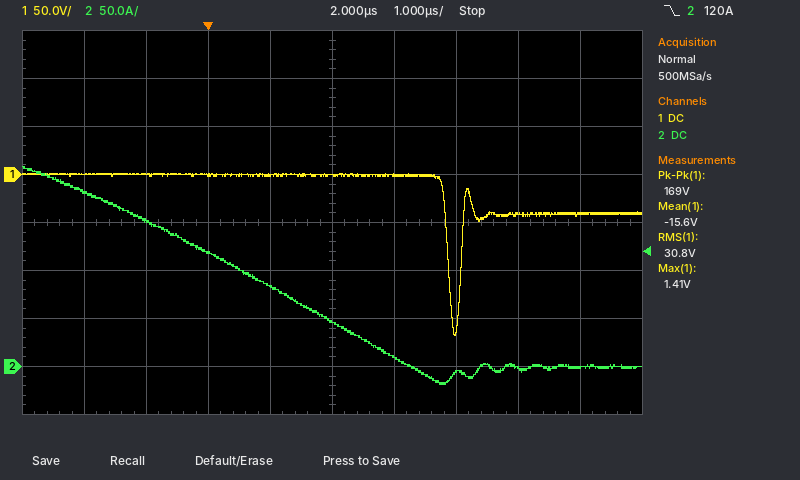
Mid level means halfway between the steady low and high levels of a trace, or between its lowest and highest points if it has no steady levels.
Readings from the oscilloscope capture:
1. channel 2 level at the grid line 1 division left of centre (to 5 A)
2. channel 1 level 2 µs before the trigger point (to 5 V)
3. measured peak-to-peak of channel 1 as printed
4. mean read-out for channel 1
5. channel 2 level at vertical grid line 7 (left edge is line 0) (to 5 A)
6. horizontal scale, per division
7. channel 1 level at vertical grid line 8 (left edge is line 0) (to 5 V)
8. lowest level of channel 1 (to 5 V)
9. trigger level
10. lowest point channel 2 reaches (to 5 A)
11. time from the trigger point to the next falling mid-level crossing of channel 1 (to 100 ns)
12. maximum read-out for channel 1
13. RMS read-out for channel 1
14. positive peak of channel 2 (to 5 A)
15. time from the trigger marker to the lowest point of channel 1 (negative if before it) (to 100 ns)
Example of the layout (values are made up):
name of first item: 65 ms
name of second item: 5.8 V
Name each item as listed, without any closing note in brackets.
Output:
channel 2 level at the grid line 1 division left of centre: 85 A
channel 1 level 2 µs before the trigger point: 0 V
measured peak-to-peak of channel 1 as printed: 169 V
mean read-out for channel 1: -15.6 V
channel 2 level at vertical grid line 7 (left edge is line 0): -5 A
horizontal scale, per division: 1 µs
channel 1 level at vertical grid line 8 (left edge is line 0): -40 V
lowest level of channel 1: -170 V
trigger level: 120 A
lowest point channel 2 reaches: -20 A
time from the trigger point to the next falling mid-level crossing of channel 1: 3.9 µs
maximum read-out for channel 1: 1.41 V
RMS read-out for channel 1: 30.8 V
positive peak of channel 2: 210 A
time from the trigger marker to the lowest point of channel 1 (negative if before it): +4.0 µs
